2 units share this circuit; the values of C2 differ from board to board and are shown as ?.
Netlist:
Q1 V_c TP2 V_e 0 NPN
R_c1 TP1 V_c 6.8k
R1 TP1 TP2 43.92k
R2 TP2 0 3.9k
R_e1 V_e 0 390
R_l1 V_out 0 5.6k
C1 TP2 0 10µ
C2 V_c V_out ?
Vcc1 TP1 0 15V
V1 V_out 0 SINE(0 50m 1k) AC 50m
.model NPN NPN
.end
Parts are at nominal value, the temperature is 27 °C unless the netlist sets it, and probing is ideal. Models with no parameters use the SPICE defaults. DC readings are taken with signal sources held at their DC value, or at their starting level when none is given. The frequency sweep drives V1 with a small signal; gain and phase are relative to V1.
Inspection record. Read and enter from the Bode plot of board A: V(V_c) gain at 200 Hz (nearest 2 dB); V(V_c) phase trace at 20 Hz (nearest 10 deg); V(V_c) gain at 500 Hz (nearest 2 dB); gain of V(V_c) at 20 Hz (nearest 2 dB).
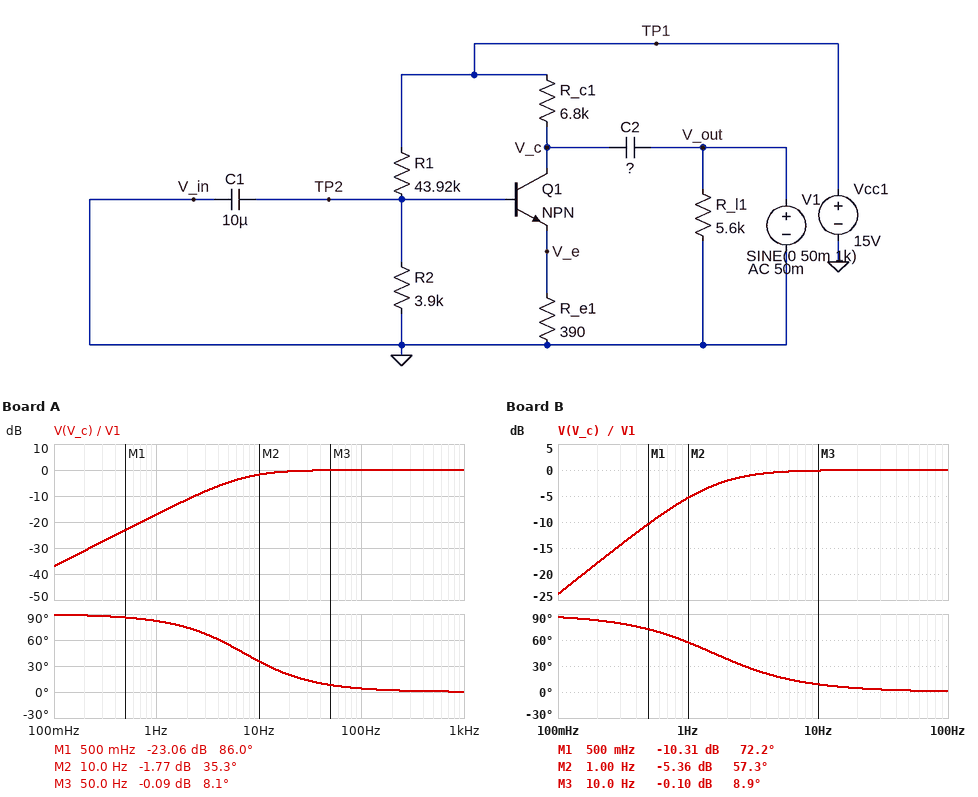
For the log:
0 dB
20 deg
0 dB
0 dB
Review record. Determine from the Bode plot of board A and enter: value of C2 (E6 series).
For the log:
3.3 µF
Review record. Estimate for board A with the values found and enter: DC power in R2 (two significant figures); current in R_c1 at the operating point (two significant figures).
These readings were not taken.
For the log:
360 µW
1.0 mA
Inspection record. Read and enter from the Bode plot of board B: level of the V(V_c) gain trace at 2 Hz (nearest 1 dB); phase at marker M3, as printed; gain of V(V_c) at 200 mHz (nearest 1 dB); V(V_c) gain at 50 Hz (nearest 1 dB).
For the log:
-2 dB
8.9 deg
-18 dB
0 dB
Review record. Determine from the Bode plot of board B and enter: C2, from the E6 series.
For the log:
15 µF
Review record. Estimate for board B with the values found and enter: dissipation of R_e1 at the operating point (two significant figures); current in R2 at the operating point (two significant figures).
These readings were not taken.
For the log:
430 µW
300 µA
